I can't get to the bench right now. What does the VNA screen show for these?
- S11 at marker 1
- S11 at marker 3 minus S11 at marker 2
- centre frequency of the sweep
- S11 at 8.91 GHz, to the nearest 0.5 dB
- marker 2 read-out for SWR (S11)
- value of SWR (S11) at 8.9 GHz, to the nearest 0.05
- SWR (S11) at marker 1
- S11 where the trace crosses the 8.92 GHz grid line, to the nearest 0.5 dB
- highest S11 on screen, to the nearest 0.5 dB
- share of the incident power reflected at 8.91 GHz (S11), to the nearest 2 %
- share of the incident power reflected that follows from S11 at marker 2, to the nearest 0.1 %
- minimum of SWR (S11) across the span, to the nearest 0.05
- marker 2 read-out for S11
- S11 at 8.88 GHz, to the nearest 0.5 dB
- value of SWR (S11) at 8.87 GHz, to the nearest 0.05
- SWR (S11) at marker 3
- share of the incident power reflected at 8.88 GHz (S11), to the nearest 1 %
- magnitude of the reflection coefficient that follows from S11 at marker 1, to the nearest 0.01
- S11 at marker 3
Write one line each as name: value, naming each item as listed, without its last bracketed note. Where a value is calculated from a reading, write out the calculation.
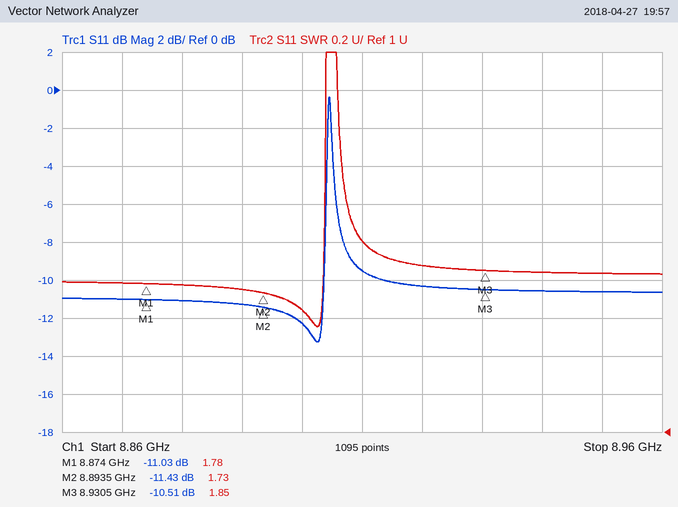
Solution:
S11 at marker 1: -11.03 dB
S11 at marker 3 minus S11 at marker 2: -10.51 − (-11.43) = 0.92 dB
centre frequency of the sweep: 8.91 GHz
S11 at 8.91 GHz, to the nearest 0.5 dB: -9.5 dB
marker 2 read-out for SWR: 1.73
value of SWR (S11) at 8.9 GHz, to the nearest 0.05: 1.65
SWR (S11) at marker 1: 1.78
S11 where the trace crosses the 8.92 GHz grid line, to the nearest 0.5 dB: -10.5 dB
highest S11 on screen, to the nearest 0.5 dB: -0.5 dB
share of the incident power reflected at 8.91 GHz (S11), to the nearest 2 %: 10^(-9.5/10) ≈ 11.2 %, so 12 % to the nearest 2 %
share of the incident power reflected that follows from S11 at marker 2, to the nearest 0.1 %: 10^(-11.43/10) ≈ 7.2 %
minimum of SWR (S11) across the span, to the nearest 0.05: 1.55
marker 2 read-out for S11: -11.43 dB
S11 at 8.88 GHz, to the nearest 0.5 dB: -11.0 dB
value of SWR (S11) at 8.87 GHz, to the nearest 0.05: 1.80
SWR (S11) at marker 3: 1.85
share of the incident power reflected at 8.88 GHz (S11), to the nearest 1 %: 10^(-11/10) ≈ 8 %
magnitude of the reflection coefficient that follows from S11 at marker 1, to the nearest 0.01: 10^(-11.03/20) ≈ 0.28
S11 at marker 3: -10.51 dB
